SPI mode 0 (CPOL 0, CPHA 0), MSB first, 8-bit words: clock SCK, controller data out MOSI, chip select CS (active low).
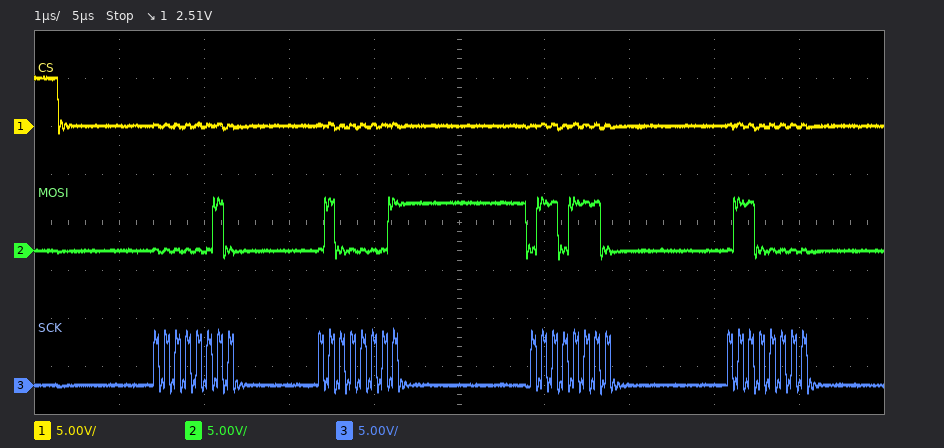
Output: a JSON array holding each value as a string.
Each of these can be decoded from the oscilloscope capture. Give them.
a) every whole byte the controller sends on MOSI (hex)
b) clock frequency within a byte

["02 41 6E 60", "8 MHz"]
